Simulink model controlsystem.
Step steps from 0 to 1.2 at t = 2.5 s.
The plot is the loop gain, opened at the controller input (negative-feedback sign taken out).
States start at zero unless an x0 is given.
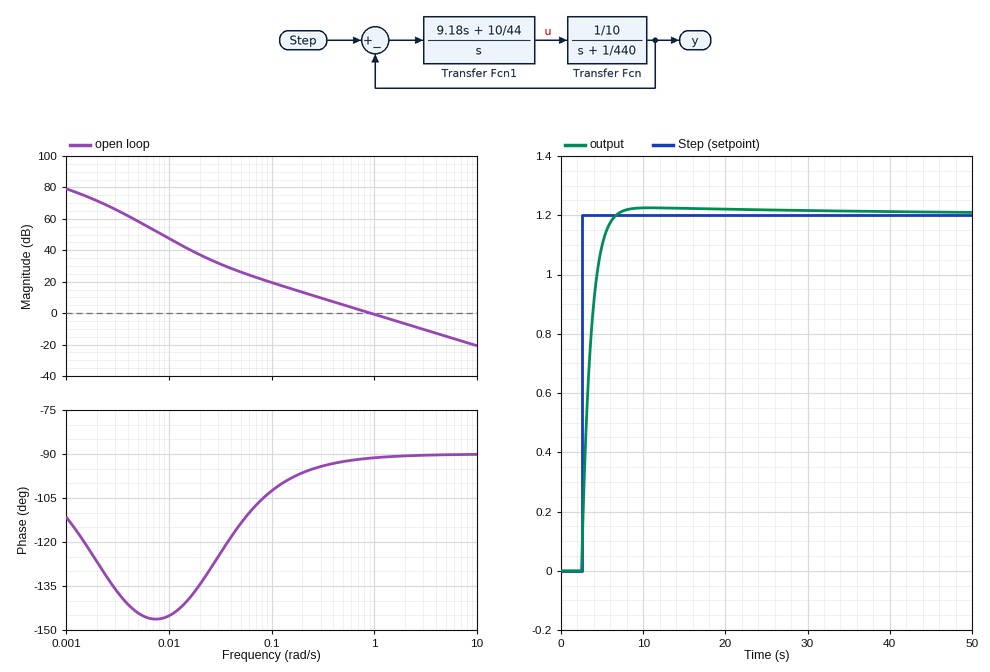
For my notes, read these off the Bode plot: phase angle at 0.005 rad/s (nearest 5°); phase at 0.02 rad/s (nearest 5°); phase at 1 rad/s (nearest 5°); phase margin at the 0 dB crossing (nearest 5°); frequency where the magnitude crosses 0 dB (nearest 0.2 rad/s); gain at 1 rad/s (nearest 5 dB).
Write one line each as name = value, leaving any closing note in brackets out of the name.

phase angle at 0.005 rad/s = -145°
phase at 0.02 rad/s = -135°
phase at 1 rad/s = -90°
phase margin at the 0 dB crossing = 90°
frequency where the magnitude crosses 0 dB = 1.0 rad/s
gain at 1 rad/s = 0 dB
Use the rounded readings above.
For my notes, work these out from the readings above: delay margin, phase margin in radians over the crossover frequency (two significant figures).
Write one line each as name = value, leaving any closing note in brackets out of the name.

delay margin, phase margin in radians over the crossover frequency = 1.6 s
